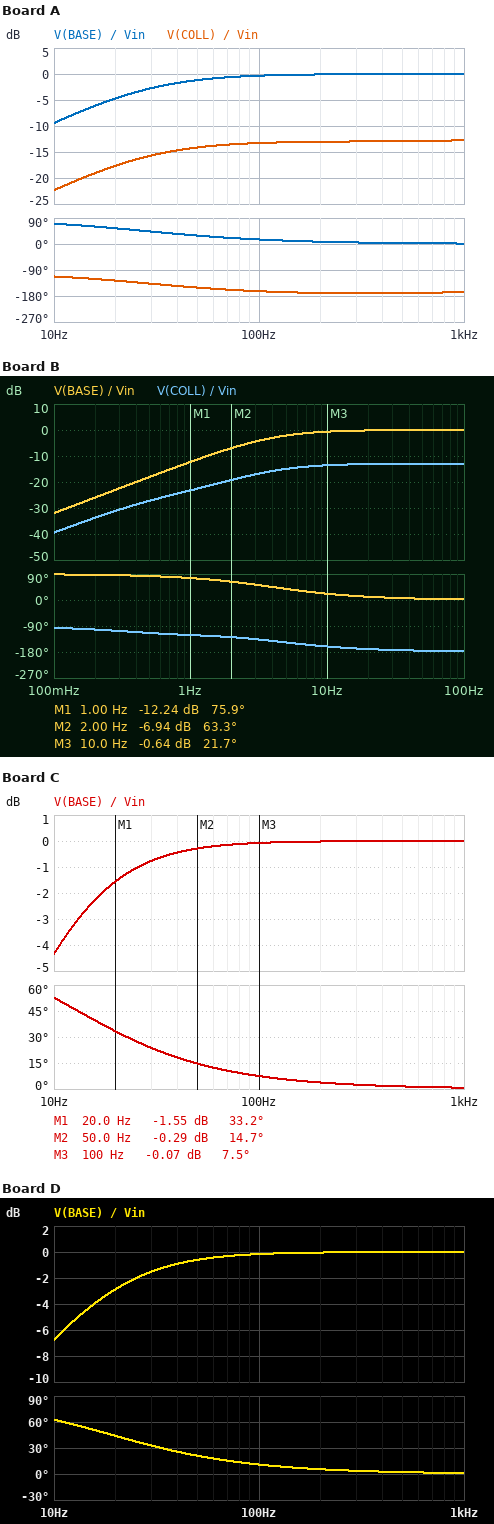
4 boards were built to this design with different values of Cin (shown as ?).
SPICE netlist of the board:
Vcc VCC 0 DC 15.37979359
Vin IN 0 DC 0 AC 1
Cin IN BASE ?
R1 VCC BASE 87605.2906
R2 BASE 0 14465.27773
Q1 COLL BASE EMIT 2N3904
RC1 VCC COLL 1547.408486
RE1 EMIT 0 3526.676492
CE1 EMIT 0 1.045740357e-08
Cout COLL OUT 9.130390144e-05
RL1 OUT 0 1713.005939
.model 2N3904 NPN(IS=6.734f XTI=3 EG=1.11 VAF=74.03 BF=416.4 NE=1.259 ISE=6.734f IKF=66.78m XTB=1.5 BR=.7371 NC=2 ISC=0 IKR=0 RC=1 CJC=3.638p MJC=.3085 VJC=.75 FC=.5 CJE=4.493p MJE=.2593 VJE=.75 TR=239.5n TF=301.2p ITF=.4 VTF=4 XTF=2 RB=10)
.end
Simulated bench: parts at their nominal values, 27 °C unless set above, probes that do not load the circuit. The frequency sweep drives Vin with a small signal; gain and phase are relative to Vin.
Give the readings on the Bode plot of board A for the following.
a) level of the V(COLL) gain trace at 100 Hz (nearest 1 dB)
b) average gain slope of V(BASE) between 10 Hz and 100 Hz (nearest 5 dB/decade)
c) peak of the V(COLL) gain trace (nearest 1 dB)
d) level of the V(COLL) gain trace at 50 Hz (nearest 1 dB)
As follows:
-13 dB
10 dB/decade
-13 dB
-14 dB
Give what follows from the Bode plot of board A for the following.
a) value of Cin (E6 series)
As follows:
470 nF
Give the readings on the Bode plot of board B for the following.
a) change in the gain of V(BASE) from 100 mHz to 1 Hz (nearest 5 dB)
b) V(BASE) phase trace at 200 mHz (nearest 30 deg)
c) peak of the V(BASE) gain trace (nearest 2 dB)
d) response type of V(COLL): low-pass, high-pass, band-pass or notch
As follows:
20 dB
90 deg
0 dB
high-pass
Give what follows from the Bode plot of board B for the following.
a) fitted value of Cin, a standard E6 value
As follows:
3.3 µF
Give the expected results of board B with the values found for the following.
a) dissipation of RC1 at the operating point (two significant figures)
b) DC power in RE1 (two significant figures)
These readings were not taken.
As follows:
280 µW
640 µW
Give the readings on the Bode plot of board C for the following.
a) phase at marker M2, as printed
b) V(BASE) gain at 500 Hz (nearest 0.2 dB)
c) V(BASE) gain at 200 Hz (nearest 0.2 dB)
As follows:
14.7 deg
0 dB
0 dB
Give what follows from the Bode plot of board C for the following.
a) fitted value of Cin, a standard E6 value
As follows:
1 µF
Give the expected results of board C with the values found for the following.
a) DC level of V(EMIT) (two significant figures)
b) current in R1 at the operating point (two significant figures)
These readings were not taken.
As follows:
1.5 V
150 µA
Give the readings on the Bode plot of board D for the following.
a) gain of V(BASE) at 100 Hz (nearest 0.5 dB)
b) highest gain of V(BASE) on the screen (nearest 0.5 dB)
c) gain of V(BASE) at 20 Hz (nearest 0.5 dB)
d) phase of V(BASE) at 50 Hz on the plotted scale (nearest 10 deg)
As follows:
0 dB
0 dB
-3.0 dB
20 deg
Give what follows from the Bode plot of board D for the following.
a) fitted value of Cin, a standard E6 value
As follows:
680 nF
